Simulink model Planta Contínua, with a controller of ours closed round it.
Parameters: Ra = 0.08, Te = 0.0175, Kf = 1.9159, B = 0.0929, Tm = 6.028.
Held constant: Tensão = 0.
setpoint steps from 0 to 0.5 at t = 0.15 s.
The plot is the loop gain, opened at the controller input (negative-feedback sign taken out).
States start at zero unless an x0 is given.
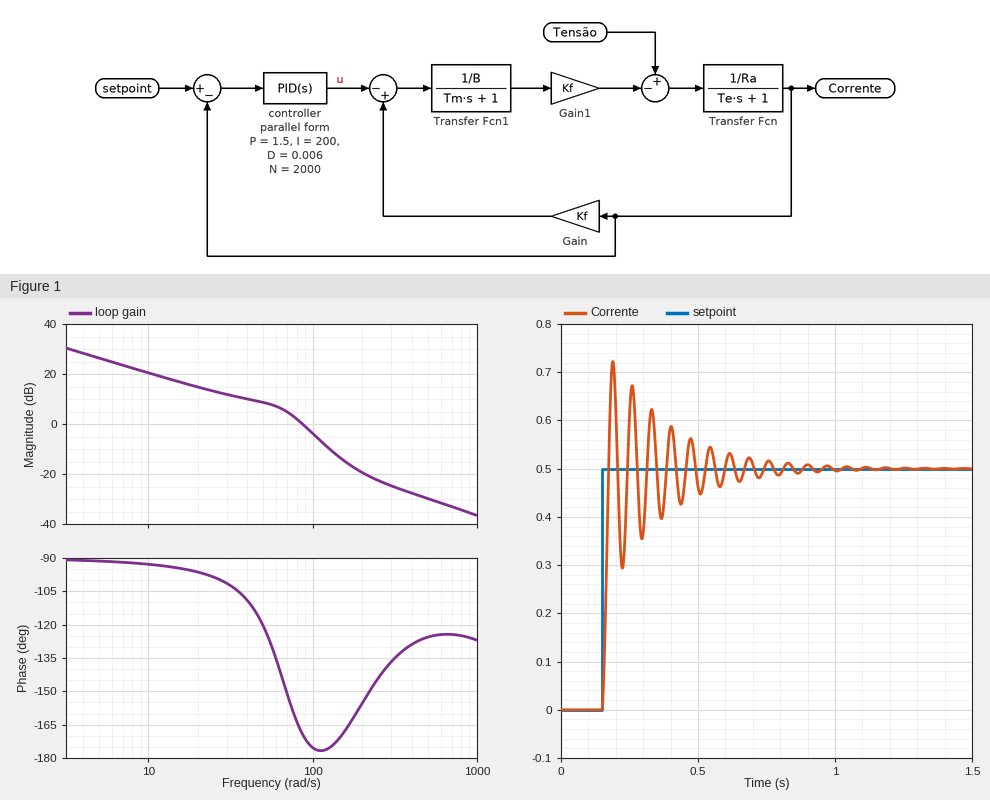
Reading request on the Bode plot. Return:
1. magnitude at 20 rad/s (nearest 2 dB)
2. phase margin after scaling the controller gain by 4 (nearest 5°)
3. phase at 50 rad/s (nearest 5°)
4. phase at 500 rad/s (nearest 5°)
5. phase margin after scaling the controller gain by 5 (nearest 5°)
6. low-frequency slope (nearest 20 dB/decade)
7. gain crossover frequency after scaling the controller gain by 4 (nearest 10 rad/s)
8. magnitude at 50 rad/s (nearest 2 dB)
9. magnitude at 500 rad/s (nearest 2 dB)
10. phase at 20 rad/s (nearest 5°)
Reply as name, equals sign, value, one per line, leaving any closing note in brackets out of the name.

magnitude at 20 rad/s = 14 dB
phase margin after scaling the controller gain by 4 = 5°
phase at 50 rad/s = -120°
phase at 500 rad/s = -125°
phase margin after scaling the controller gain by 5 = 10°
low-frequency slope = -20 dB/decade
gain crossover frequency after scaling the controller gain by 4 = 140 rad/s
magnitude at 50 rad/s = 8 dB
magnitude at 500 rad/s = -30 dB
phase at 20 rad/s = -95°
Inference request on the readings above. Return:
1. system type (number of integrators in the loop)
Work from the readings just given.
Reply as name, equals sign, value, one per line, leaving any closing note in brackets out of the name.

system type = 1
